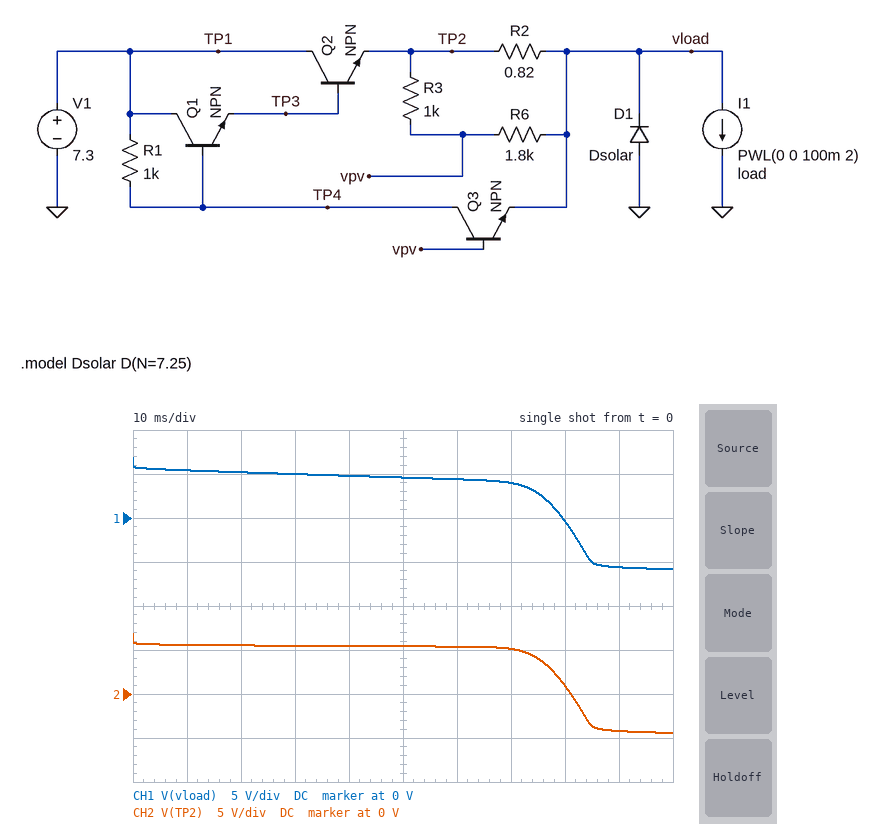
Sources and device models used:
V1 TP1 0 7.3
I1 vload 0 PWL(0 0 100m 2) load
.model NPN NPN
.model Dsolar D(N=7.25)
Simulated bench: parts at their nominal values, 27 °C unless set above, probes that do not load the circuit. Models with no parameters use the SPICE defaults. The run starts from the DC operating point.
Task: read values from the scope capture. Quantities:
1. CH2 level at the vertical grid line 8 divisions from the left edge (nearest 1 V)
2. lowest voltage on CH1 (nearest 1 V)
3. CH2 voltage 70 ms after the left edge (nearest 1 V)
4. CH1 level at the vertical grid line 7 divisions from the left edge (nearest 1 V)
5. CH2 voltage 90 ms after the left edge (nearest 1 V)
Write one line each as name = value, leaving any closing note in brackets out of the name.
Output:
CH2 level at the vertical grid line 8 divisions from the left edge = 1 V
lowest voltage on CH1 = -6 V
CH2 voltage 70 ms after the left edge = 5 V
CH1 level at the vertical grid line 7 divisions from the left edge = 4 V
CH2 voltage 90 ms after the left edge = -4 V
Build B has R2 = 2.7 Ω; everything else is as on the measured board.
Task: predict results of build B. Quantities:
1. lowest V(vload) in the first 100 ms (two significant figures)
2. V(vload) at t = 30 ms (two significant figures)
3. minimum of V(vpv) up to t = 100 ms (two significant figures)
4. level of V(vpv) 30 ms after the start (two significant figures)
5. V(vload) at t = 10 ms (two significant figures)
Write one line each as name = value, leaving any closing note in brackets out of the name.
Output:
lowest V(vload) in the first 100 ms = -6.1 V
V(vload) at t = 30 ms = -5.6 V
minimum of V(vpv) up to t = 100 ms = -5.3 V
level of V(vpv) 30 ms after the start = -4.7 V
V(vload) at t = 10 ms = 5.0 V
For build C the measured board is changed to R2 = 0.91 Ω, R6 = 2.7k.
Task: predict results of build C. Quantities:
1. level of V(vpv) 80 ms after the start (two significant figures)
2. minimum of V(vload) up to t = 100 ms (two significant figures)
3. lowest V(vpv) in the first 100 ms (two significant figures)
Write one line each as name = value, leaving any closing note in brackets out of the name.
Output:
level of V(vpv) 80 ms after the start = -4.9 V
minimum of V(vload) up to t = 100 ms = -6.0 V
lowest V(vpv) in the first 100 ms = -5.1 V
